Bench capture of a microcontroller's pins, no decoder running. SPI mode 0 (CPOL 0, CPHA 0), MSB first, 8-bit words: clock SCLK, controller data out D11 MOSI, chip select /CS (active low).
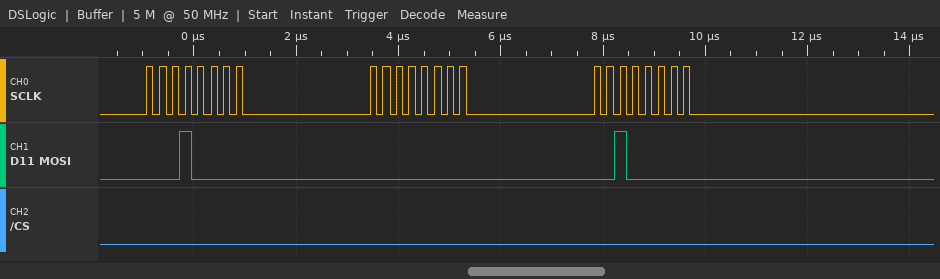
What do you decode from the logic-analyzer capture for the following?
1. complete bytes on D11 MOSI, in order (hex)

0x10 0x00 0x20
